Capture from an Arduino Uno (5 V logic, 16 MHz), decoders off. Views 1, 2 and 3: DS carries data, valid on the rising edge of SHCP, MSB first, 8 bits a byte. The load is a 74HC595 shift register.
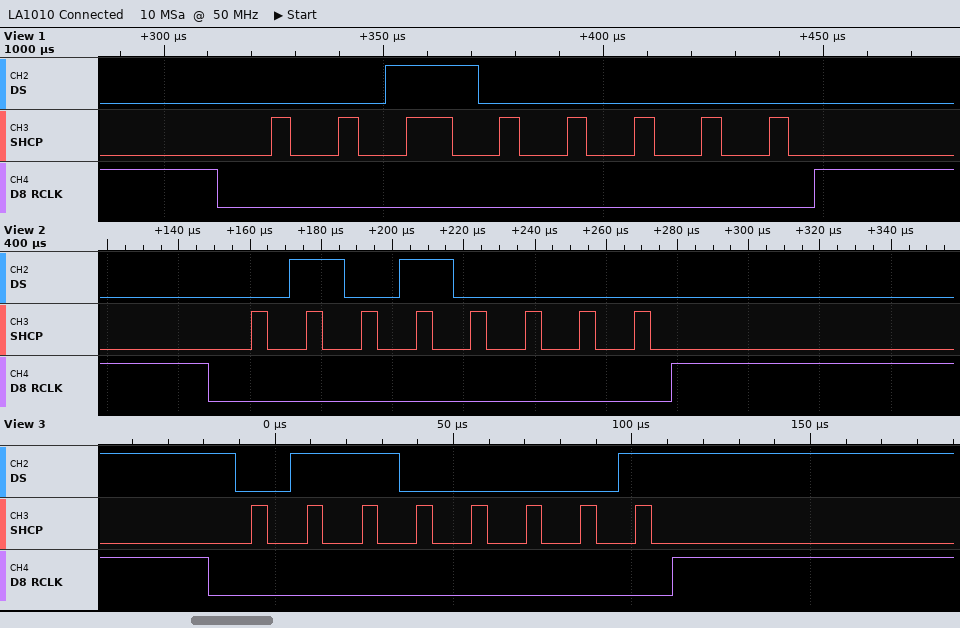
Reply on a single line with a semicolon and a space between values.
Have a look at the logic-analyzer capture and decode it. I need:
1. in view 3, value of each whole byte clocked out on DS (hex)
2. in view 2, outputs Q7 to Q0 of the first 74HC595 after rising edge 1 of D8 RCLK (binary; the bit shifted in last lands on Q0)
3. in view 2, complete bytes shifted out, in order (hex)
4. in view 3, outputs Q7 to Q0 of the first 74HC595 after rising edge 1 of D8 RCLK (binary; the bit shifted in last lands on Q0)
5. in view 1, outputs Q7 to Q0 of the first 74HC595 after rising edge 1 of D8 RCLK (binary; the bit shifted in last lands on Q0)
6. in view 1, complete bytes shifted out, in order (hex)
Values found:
61; 01010000; 50; 01100001; 00100000; 20
